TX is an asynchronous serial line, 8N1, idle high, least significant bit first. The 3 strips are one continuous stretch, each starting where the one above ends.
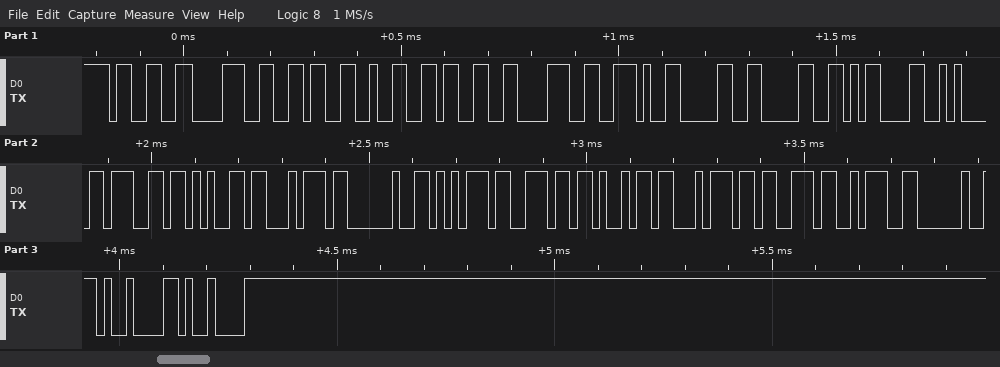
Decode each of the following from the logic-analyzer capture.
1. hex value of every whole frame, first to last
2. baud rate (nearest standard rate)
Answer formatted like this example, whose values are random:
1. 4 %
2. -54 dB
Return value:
1. 0x33 0x38 0x36 0x32 0x33 0x38 0x2E 0x30 0x30 0x0D 0x0A 0x67 0x65 0x74 0x20 0x75 0x6E 0x69 0x74 0x73 0x3A 0x20 0x09 0x09
2. 57600 baud
